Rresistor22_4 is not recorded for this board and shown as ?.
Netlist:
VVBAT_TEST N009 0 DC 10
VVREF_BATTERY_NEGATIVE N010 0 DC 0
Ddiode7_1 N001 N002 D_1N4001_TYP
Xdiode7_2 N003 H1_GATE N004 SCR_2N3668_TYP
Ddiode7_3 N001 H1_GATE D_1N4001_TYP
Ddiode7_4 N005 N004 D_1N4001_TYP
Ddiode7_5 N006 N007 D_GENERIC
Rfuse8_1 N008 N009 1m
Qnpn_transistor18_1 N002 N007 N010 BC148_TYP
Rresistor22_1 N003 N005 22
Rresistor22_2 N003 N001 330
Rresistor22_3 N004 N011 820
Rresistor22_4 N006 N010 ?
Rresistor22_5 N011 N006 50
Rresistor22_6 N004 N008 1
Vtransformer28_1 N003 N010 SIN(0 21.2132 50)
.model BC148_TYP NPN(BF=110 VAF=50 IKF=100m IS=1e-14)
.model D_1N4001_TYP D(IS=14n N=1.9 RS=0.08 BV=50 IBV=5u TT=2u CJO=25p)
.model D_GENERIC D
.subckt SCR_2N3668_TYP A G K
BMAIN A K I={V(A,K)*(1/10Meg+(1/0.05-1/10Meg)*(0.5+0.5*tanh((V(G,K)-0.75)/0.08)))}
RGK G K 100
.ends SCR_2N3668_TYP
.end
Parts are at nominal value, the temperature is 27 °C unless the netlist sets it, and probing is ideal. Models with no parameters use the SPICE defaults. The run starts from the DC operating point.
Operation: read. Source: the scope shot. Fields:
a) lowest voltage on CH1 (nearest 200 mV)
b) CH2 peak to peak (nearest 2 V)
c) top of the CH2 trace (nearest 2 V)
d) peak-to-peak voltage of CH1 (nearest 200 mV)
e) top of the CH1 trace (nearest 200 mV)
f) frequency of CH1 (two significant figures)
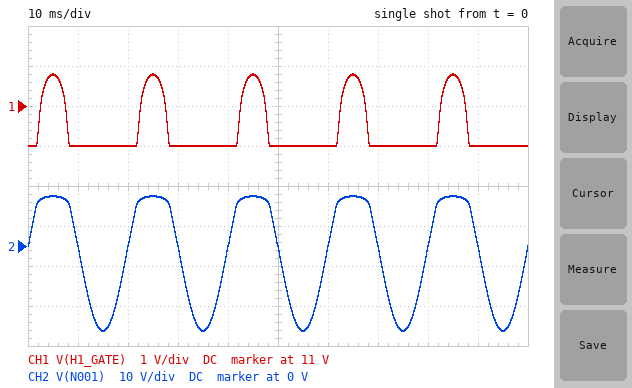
10.0 V
34 V
12 V
1.8 V
11.8 V
50 Hz
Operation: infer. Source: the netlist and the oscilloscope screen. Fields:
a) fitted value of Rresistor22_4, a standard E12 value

120 Ω
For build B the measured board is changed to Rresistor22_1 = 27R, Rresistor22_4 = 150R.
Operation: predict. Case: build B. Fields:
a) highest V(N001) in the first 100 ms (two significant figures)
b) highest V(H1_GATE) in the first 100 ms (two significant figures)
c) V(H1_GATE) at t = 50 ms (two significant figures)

2.3 V
10 V
10 V
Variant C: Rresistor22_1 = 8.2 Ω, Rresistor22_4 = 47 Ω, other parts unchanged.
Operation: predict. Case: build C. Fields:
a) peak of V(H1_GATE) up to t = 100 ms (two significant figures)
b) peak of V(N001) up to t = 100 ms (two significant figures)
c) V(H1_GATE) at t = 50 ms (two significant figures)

18 V
19 V
10 V
